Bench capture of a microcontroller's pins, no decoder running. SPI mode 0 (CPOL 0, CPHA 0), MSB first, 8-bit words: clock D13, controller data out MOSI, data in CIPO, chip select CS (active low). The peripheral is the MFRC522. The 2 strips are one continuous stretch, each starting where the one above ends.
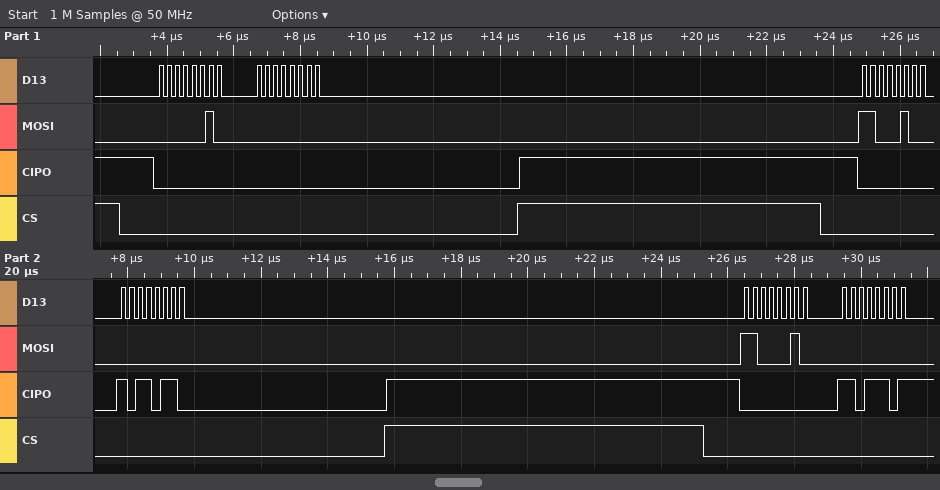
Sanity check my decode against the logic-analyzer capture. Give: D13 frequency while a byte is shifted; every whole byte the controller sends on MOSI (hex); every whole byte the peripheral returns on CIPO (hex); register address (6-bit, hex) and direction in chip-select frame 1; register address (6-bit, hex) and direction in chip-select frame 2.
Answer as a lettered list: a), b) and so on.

a) 4 MHz
b) 02 00 C4 00 C2 00
c) 00 00 00 B6 00 DD
d) 0x01 write
e) 0x22 read
